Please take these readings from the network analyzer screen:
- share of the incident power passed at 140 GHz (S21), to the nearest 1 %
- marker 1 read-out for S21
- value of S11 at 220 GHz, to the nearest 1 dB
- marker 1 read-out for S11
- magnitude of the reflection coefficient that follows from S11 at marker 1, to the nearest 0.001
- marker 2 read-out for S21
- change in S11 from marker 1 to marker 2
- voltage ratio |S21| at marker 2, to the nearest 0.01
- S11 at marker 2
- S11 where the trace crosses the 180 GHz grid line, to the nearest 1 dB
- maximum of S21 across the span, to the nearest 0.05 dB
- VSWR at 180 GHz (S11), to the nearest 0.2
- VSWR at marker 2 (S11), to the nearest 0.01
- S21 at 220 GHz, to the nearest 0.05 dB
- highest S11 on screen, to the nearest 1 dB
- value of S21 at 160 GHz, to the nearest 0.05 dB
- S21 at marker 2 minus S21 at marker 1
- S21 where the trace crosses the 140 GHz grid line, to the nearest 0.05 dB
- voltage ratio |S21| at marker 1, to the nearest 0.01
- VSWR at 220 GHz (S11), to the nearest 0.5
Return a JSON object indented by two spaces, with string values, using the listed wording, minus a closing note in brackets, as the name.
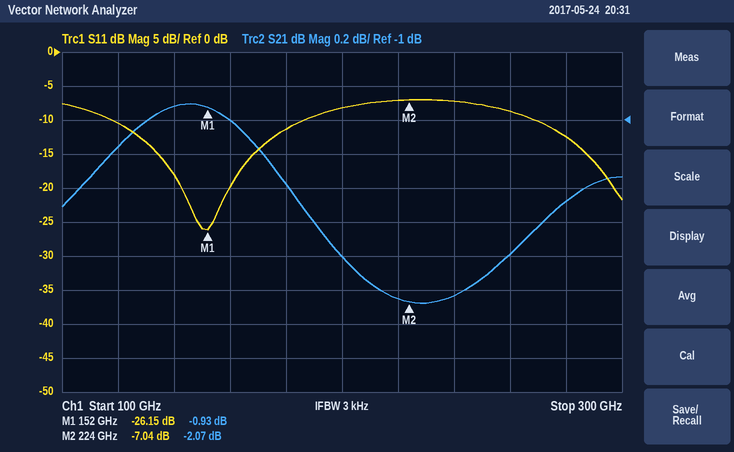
{
  "share of the incident power passed at 140 GHz (S21), to the nearest 1 %": "81 %",
  "marker 1 read-out for S21": "-0.93 dB",
  "value of S11 at 220 GHz, to the nearest 1 dB": "-7 dB",
  "marker 1 read-out for S11": "-26.15 dB",
  "magnitude of the reflection coefficient that follows from S11 at marker 1, to the nearest 0.001": "0.049",
  "marker 2 read-out for S21": "-2.07 dB",
  "change in S11 from marker 1 to marker 2": "19.11 dB",
  "voltage ratio |S21| at marker 2, to the nearest 0.01": "0.79",
  "S11 at marker 2": "-7.04 dB",
  "S11 where the trace crosses the 180 GHz grid line, to the nearest 1 dB": "-11 dB",
  "maximum of S21 across the span, to the nearest 0.05 dB": "-0.90 dB",
  "VSWR at 180 GHz (S11), to the nearest 0.2": "1.8",
  "VSWR at marker 2 (S11), to the nearest 0.01": "2.60",
  "S21 at 220 GHz, to the nearest 0.05 dB": "-2.05 dB",
  "highest S11 on screen, to the nearest 1 dB": "-7 dB",
  "value of S21 at 160 GHz, to the nearest 0.05 dB": "-1.00 dB",
  "S21 at marker 2 minus S21 at marker 1": "-1.14 dB",
  "S21 where the trace crosses the 140 GHz grid line, to the nearest 0.05 dB": "-0.90 dB",
  "voltage ratio |S21| at marker 1, to the nearest 0.01": "0.90",
  "VSWR at 220 GHz (S11), to the nearest 0.5": "2.5"
}
